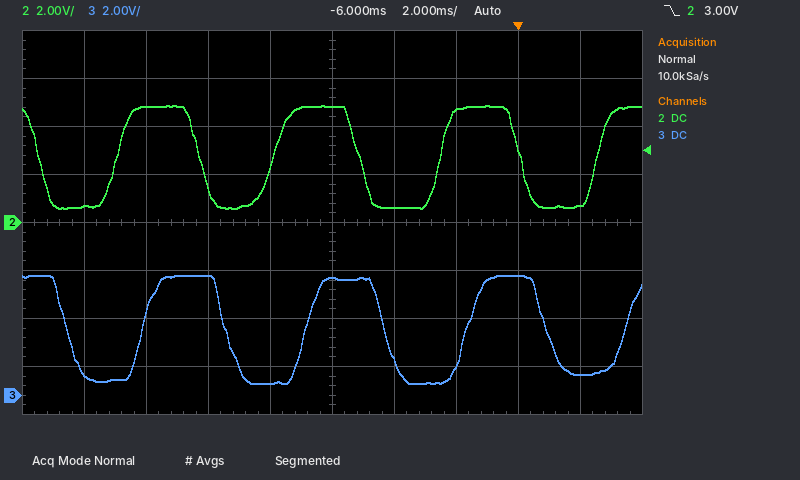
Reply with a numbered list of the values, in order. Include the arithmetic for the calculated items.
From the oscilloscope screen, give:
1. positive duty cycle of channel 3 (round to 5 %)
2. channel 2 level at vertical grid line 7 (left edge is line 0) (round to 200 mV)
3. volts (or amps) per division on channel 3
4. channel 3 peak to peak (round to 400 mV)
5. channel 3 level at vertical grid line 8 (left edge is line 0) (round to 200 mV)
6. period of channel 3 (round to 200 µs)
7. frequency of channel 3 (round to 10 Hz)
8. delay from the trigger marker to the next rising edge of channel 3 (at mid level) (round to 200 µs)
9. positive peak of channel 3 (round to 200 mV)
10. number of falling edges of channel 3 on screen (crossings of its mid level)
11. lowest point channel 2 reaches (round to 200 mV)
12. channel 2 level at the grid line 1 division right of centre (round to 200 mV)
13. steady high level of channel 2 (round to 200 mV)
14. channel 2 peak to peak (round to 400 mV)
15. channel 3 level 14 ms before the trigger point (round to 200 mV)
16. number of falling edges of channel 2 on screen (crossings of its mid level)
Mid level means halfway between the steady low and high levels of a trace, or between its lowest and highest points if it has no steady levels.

1. 50 %
2. 4.6 V
3. 2 V
4. 4.4 V
5. 5.0 V
6. 5.2 ms
7. 1 / 5.2 ms ≈ 192 Hz, so 190 Hz to the nearest 10 Hz
8. 3.4 ms
9. 5.0 V
10. 4
11. 600 mV
12. 600 mV
13. 4.8 V
14. 4.4 V
15. 800 mV
16. 4
